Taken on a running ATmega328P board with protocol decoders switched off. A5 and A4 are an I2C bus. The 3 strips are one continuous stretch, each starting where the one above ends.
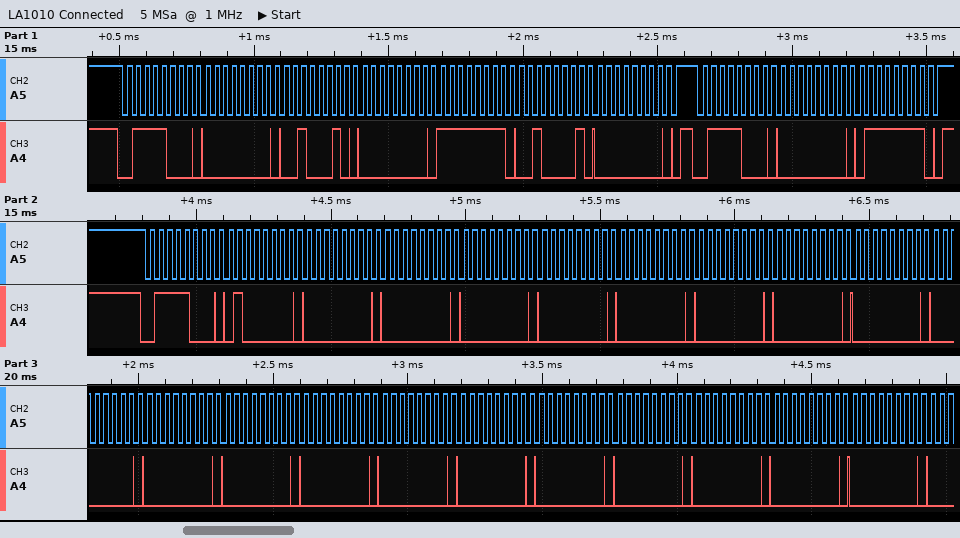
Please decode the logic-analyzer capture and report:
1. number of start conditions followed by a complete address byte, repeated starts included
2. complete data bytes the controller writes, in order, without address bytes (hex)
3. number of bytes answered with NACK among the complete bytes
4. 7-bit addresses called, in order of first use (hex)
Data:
3
00 22 00 FF 21 00 00 7F 40 00 00 00 00 00 00 00 00 00 00 00 00 00 00 00 00 00 00 00
0
0x3C
